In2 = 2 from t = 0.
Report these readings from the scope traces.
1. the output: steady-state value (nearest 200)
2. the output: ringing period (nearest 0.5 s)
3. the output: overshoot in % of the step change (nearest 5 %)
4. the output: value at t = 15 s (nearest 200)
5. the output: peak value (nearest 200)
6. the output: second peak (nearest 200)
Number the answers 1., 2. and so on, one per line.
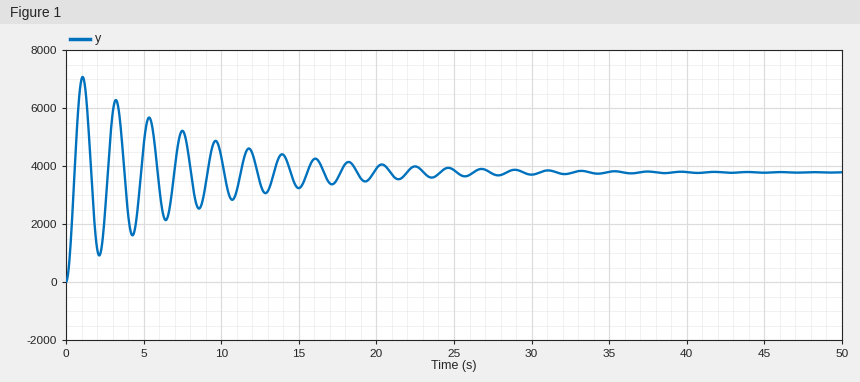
1. 3800
2. 2.0 s
3. 85 %
4. 3200
5. 7000
6. 6200
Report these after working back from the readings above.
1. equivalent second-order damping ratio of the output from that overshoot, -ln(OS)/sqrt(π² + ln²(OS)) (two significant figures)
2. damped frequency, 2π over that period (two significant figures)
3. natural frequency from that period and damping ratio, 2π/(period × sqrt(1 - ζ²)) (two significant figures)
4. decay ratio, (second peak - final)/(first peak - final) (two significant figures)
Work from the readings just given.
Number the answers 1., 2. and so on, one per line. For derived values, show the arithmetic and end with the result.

1. ln(0.85) = -0.163; 0.163 / sqrt(9.870 + 0.026) = 0.052
2. 2π / 2 = 3.1 rad/s
3. 2π / (2 × sqrt(1 - 0.052²)) = 3.1 rad/s
4. (6200 - 3800) / (7000 - 3800) = 0.75
